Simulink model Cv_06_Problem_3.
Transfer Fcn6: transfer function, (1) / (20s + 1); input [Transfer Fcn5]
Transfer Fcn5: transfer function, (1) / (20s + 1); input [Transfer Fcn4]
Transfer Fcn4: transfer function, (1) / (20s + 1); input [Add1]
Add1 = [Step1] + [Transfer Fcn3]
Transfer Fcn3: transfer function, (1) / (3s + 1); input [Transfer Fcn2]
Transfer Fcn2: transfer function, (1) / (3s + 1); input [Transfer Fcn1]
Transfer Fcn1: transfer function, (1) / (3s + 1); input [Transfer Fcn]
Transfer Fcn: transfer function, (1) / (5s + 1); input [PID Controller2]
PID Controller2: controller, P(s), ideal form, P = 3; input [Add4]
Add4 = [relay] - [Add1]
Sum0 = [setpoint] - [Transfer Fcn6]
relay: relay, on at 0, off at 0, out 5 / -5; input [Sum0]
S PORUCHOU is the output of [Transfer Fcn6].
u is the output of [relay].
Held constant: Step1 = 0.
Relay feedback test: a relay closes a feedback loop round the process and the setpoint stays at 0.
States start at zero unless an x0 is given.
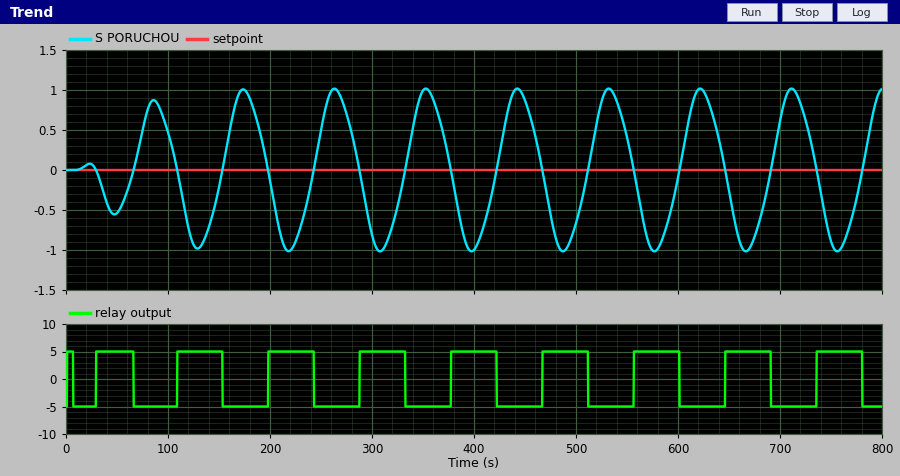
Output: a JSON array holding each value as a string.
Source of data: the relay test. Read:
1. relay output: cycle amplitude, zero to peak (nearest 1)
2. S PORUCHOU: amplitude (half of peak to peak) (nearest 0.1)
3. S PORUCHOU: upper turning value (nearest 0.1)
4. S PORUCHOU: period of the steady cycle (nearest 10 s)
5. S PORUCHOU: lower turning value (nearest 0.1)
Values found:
["5", "1.0", "1.0", "90 s", "-1.0"]
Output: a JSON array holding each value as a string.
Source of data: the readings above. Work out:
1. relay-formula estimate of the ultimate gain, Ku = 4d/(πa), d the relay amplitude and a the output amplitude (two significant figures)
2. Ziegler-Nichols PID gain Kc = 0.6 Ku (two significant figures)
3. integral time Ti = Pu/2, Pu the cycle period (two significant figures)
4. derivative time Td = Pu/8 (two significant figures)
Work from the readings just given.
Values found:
["6.4", "3.8", "45 s", "11 s"]
